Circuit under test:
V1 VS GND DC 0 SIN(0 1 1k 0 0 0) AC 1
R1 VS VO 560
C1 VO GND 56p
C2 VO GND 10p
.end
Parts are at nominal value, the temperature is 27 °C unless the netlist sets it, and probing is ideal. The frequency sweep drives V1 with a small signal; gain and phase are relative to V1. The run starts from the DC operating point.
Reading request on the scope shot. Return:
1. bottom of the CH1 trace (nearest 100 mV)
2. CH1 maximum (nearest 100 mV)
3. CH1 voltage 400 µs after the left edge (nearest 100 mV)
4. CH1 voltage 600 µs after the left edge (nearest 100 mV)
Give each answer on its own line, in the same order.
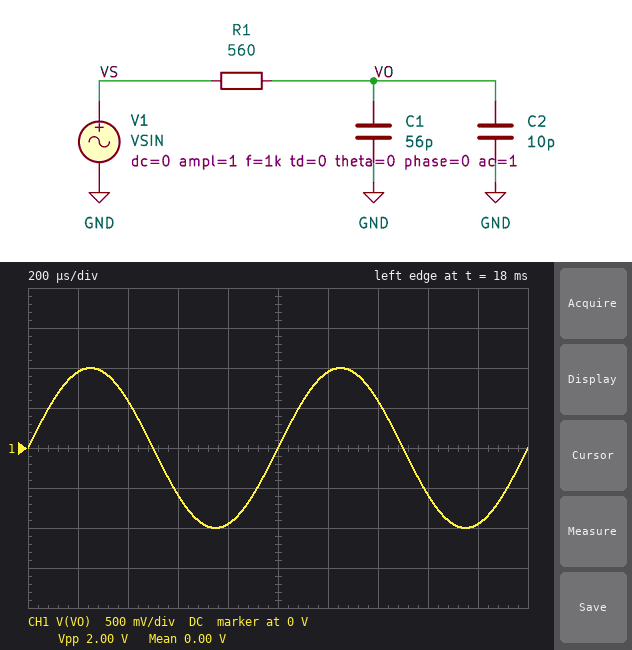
-1.0 V
1.0 V
600 mV
-600 mV
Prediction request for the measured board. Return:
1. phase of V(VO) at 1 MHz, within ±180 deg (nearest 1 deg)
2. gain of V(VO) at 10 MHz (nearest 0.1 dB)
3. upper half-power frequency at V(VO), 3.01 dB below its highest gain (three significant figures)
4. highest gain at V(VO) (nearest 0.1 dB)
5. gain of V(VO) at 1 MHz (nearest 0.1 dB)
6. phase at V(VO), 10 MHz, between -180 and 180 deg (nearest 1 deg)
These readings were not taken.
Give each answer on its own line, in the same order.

-13 deg
-8.1 dB
4.31 MHz
0 dB
-0.2 dB
-67 deg
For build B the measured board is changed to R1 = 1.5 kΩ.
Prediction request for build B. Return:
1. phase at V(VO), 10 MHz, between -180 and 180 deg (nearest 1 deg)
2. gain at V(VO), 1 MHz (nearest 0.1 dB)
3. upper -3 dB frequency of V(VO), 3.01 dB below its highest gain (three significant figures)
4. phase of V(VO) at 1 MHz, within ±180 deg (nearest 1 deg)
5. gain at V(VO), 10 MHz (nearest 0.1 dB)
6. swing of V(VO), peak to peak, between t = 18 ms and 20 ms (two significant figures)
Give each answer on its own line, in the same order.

-81 deg
-1.4 dB
1.61 MHz
-32 deg
-16.0 dB
2.0 V
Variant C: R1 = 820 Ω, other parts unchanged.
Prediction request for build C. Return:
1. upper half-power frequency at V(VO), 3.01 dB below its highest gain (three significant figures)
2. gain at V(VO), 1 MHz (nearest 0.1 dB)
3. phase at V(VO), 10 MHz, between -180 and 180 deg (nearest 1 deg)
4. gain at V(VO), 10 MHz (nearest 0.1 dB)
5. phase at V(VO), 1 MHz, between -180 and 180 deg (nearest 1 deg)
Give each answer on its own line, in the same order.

2.94 MHz
-0.5 dB
-74 deg
-11.0 dB
-19 deg
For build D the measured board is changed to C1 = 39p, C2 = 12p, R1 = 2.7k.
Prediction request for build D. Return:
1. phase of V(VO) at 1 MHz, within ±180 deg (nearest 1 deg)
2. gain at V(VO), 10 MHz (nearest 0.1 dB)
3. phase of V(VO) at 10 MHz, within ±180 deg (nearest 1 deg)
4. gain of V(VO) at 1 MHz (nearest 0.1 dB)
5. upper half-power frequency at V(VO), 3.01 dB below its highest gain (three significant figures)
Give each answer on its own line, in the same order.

-41 deg
-18.8 dB
-83 deg
-2.4 dB
1.16 MHz
